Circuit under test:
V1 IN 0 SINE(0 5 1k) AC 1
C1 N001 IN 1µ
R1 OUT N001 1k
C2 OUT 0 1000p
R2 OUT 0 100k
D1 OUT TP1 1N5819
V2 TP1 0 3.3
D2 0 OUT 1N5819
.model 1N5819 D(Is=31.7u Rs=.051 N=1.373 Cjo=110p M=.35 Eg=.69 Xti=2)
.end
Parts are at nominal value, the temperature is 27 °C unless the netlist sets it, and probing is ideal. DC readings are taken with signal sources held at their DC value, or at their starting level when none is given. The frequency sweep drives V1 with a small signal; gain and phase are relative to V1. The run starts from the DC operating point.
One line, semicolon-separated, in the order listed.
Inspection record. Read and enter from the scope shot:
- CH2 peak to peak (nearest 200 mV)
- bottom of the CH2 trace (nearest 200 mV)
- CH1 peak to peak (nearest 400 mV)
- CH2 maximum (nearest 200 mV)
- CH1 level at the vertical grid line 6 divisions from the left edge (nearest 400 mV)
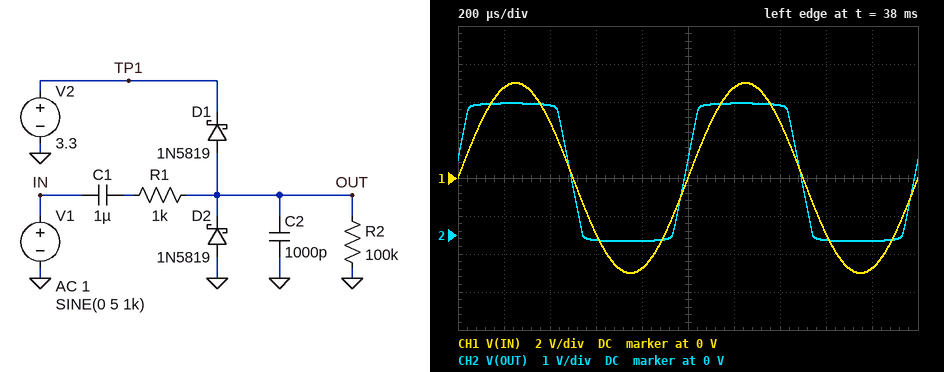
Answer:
3.6 V; -200 mV; 10.0 V; 3.4 V; 4.8 V
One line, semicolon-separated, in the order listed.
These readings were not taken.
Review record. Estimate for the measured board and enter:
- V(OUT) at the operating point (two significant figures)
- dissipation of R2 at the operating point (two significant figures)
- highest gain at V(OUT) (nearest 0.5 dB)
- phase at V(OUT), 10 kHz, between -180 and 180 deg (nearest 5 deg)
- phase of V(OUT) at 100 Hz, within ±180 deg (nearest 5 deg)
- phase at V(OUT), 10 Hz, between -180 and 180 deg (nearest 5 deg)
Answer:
120 mV; 140 nW; -0.5 dB; -5 deg; 5 deg; 30 deg
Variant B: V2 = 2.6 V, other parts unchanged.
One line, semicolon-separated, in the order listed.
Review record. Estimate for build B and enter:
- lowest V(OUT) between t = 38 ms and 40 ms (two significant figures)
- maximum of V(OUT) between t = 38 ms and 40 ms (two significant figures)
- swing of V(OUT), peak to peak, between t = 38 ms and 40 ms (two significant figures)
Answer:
-170 mV; 2.8 V; 2.9 V
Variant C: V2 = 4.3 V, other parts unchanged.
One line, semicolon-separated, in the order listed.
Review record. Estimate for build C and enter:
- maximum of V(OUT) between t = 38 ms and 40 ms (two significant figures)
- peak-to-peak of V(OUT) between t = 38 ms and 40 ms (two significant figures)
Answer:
4.5 V; 4.6 V
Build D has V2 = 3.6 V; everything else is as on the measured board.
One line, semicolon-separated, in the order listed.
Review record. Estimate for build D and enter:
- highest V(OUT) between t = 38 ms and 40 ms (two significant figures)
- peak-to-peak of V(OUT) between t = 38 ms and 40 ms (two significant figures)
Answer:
3.8 V; 3.9 V
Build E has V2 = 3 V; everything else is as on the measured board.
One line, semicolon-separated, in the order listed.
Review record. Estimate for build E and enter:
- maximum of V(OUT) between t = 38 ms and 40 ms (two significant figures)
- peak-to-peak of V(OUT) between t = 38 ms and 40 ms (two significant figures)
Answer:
3.2 V; 3.3 V
